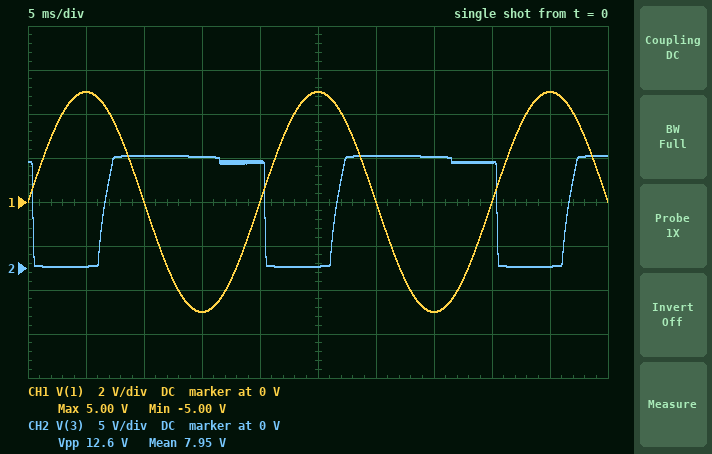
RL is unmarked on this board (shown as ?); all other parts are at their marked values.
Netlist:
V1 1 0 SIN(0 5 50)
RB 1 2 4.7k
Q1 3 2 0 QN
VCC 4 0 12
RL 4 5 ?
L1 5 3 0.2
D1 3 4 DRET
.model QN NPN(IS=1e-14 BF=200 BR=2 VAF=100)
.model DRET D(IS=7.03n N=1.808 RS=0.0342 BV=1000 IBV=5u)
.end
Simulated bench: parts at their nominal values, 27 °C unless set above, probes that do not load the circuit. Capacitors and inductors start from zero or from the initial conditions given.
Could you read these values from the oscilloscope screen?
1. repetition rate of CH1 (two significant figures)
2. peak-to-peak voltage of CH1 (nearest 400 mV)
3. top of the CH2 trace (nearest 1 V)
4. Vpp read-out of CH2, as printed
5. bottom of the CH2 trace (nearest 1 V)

50 Hz
10.0 V
13 V
12.6 V
0 V
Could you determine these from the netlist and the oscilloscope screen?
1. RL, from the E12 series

56 Ω
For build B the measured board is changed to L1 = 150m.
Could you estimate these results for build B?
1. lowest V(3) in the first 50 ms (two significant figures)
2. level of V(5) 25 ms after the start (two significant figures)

180 mV
2.4 V
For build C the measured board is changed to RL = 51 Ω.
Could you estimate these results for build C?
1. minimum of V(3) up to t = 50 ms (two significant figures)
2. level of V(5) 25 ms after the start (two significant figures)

160 mV
3.9 V
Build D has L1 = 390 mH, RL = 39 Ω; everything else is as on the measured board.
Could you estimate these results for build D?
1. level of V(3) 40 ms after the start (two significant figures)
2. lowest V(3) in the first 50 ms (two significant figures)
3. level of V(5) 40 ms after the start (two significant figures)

13 V
120 mV
11 V
